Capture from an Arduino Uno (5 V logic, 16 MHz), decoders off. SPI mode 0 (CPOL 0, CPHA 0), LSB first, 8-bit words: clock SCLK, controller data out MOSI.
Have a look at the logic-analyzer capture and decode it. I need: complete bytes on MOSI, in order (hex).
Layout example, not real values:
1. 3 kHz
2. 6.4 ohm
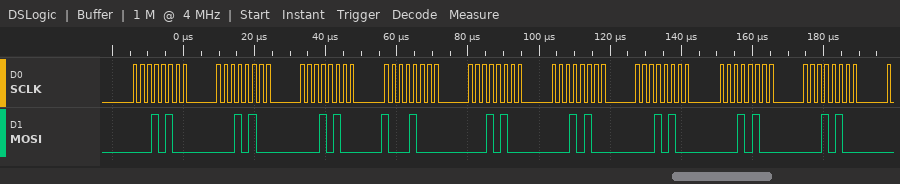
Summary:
1. 28 28 28 11 28 28 28 28 28
